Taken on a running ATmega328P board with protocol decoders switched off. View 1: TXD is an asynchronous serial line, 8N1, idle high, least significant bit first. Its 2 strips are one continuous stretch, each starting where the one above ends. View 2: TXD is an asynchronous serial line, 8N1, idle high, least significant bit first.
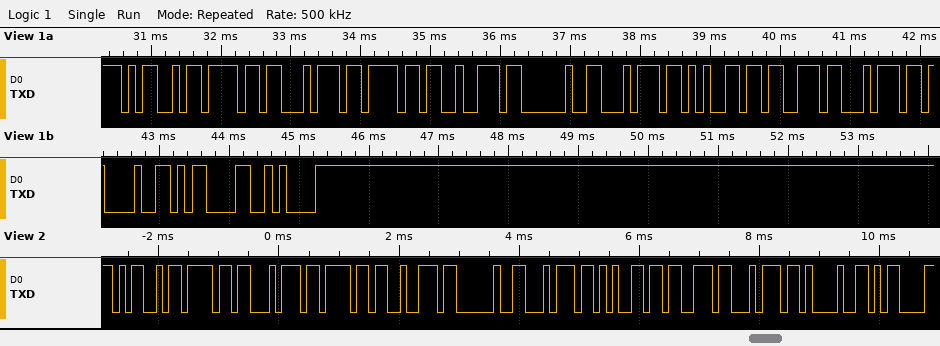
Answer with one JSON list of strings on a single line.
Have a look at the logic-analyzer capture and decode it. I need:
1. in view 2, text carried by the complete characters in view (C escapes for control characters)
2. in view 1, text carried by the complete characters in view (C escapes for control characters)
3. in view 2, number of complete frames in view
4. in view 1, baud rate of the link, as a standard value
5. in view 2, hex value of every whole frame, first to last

["\"Motor test!\\r\"", "\"Motor test!\\r\\n\"", "12", "9600 baud", "4D 6F 74 6F 72 20 74 65 73 74 21 0D"]
